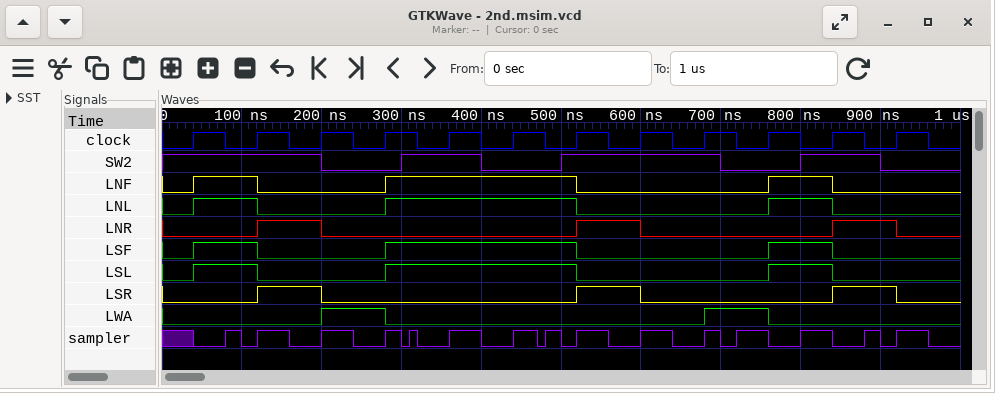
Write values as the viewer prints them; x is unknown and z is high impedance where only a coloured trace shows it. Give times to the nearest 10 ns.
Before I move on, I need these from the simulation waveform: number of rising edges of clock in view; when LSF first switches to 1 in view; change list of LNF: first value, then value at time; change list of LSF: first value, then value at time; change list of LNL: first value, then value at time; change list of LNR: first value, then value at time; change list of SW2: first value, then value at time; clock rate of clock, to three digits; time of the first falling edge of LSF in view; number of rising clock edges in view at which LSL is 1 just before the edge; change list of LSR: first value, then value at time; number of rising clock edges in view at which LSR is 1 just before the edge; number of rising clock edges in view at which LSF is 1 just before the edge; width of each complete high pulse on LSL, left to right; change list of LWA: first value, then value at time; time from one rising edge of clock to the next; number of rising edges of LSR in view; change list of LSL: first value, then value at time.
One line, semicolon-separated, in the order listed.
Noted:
12; 40 ns; 0, 1 at 40 ns, 0 at 120 ns, 1 at 280 ns, 0 at 520 ns, 1 at 760 ns, 0 at 840 ns; 0, 1 at 40 ns, 0 at 120 ns, 1 at 280 ns, 0 at 520 ns, 1 at 760 ns, 0 at 840 ns; 0, 1 at 40 ns, 0 at 120 ns, 1 at 280 ns, 0 at 520 ns, 1 at 760 ns, 0 at 840 ns; 0, 1 at 120 ns, 0 at 200 ns, 1 at 520 ns, 0 at 600 ns, 1 at 840 ns, 0 at 920 ns; 1, 0 at 200 ns, 1 at 300 ns, 0 at 400 ns, 1 at 500 ns, 0 at 700 ns, 1 at 800 ns, 0 at 900 ns; 12.5 MHz; 120 ns; 5; 0, 1 at 120 ns, 0 at 200 ns, 1 at 520 ns, 0 at 600 ns, 1 at 840 ns, 0 at 920 ns; 3; 5; 80 ns, 240 ns, 80 ns; 0, 1 at 200 ns, 0 at 280 ns, 1 at 680 ns, 0 at 760 ns; 80 ns; 3; 0, 1 at 40 ns, 0 at 120 ns, 1 at 280 ns, 0 at 520 ns, 1 at 760 ns, 0 at 840 ns
